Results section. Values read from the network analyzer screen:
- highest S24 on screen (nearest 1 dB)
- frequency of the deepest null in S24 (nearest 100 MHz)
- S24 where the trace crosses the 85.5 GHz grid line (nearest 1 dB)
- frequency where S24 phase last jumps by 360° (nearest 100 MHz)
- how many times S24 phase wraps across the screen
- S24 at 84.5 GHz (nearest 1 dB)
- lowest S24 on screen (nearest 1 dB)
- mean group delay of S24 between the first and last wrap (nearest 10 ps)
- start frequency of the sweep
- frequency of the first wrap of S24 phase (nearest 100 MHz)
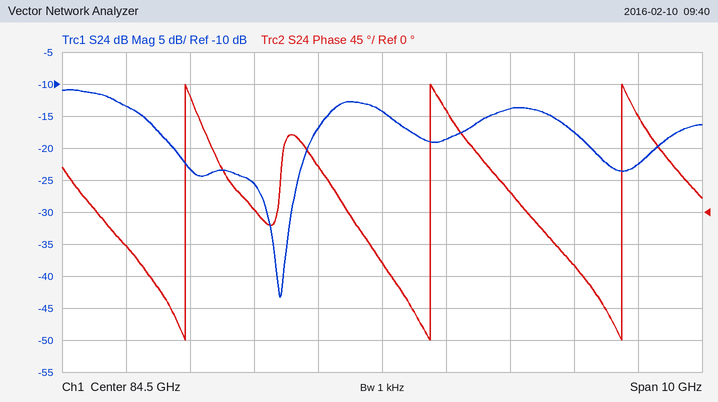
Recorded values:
-11 dB
82.9 GHz
-19 dB
88.2 GHz
3
-14 dB
-43 dB
290 ps
79.5 GHz
81.4 GHz
